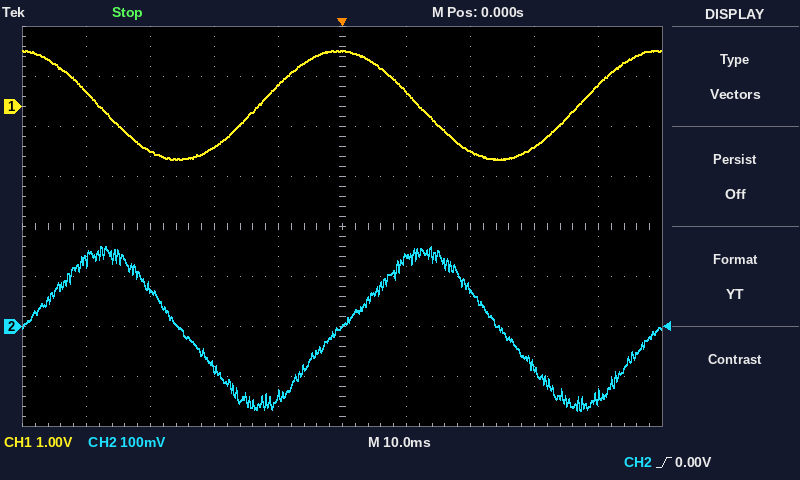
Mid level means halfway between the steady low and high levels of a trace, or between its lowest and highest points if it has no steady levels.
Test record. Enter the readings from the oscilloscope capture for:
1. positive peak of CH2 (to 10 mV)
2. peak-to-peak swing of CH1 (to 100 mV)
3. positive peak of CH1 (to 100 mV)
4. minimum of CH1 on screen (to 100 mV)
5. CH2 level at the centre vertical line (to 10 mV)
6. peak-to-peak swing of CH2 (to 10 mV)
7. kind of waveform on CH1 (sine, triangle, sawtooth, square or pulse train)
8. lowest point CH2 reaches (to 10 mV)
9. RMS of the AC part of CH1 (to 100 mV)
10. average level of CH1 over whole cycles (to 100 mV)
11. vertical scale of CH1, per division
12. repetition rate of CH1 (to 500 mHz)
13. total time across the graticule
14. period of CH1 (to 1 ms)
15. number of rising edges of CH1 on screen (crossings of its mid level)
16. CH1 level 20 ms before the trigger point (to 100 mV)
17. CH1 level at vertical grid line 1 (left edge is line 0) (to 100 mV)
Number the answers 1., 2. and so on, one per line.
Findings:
1. 160 mV
2. 2.2 V
3. 1.1 V
4. -1.1 V
5. 0 mV
6. 330 mV
7. sine
8. -170 mV
9. 800 mV
10. 0.0 V
11. 1 V
12. 20.0 Hz
13. 100 ms
14. 50 ms
15. 2
16. -800 mV
17. 300 mV
